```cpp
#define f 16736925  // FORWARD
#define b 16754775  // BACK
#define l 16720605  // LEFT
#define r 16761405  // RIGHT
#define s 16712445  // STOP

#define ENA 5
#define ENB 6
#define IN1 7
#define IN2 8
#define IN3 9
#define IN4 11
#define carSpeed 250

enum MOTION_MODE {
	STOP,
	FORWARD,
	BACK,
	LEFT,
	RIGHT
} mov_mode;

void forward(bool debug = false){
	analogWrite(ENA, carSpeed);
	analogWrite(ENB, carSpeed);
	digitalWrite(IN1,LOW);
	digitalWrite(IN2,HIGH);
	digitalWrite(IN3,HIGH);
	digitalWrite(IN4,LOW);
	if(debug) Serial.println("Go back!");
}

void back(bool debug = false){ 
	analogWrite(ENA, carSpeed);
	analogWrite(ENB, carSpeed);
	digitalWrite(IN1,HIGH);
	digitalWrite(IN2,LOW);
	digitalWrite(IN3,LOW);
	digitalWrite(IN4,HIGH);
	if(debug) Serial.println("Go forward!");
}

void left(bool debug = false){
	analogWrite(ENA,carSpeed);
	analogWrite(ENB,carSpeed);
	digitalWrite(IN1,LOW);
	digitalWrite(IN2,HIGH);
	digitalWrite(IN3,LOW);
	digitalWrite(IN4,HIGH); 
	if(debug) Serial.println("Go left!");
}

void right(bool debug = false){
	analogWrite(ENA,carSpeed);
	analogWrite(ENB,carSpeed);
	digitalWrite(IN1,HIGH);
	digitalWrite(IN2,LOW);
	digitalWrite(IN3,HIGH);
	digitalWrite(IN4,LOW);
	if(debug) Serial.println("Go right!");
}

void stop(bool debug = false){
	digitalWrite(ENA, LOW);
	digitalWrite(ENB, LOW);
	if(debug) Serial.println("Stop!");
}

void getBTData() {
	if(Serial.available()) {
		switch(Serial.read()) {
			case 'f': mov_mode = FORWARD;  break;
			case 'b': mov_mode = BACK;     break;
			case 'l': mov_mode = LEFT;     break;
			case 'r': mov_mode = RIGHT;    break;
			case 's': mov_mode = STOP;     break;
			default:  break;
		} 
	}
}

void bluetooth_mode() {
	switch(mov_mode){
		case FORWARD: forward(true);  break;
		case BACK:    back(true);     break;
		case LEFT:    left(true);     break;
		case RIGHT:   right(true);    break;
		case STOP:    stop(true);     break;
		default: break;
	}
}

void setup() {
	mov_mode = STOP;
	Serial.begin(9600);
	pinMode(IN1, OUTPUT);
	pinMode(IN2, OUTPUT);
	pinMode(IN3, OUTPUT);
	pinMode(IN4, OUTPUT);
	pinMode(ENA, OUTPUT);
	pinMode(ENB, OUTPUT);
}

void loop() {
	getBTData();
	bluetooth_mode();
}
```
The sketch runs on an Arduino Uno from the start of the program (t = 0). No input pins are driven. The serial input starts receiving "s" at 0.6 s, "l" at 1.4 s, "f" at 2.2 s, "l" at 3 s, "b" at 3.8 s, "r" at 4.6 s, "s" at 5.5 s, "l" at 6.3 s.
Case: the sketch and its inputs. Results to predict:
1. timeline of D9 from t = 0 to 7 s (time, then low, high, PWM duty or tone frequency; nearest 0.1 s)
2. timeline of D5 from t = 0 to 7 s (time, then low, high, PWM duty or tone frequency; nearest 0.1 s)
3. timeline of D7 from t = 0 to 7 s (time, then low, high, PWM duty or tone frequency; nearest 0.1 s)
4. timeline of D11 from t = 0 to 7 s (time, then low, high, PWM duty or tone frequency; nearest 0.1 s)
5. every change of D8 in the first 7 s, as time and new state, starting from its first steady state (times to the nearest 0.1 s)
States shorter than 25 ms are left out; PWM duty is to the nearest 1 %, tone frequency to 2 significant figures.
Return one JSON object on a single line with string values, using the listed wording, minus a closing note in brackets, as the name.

{"timeline of D9 from t = 0 to 7 s": "0 s low; 2.2 s high; 3 s low; 4.6 s high; 6.3 s low", "timeline of D5 from t = 0 to 7 s": "0 s low; 1.4 s PWM 98 %; 5.5 s low; 6.3 s PWM 98 %", "timeline of D7 from t = 0 to 7 s": "0 s low; 3.8 s high; 6.3 s low", "timeline of D11 from t = 0 to 7 s": "0 s low; 1.4 s high; 2.2 s low; 3 s high; 4.6 s low; 6.3 s high", "every change of D8 in the first 7 s, as time and new state, starting from its first steady state": "0 s low; 1.4 s high; 3.8 s low; 6.3 s high"}
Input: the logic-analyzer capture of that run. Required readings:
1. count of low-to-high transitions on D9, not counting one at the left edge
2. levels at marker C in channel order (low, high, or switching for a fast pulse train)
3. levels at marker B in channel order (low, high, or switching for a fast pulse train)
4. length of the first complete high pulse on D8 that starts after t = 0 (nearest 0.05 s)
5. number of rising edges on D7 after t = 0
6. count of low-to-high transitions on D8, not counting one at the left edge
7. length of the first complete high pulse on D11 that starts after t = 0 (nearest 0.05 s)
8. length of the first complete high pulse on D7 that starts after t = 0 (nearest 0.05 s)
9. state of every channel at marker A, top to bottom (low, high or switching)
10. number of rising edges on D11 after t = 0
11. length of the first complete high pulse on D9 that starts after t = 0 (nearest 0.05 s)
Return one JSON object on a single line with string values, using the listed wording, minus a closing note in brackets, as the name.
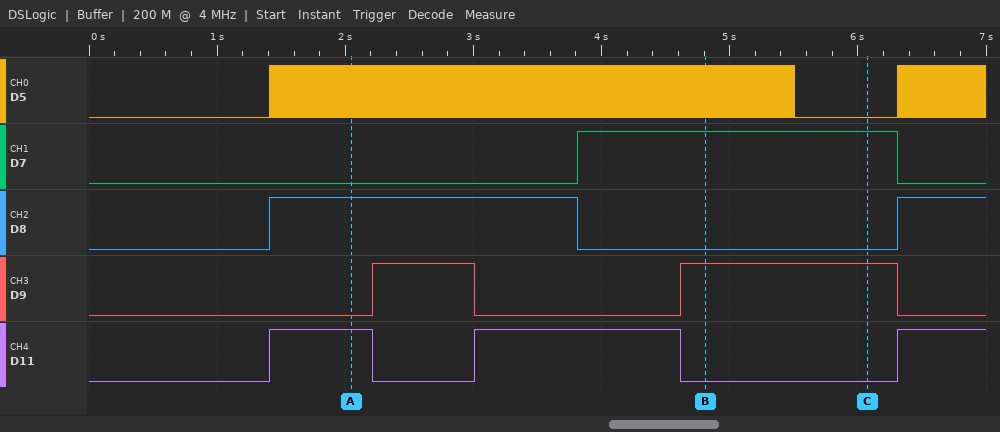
{"count of low-to-high transitions on D9, not counting one at the left edge": "2", "levels at marker C in channel order": "D5 low, D7 high, D8 low, D9 high, D11 low", "levels at marker B in channel order": "D5 switching, D7 high, D8 low, D9 high, D11 low", "length of the first complete high pulse on D8 that starts after t = 0": "2.40 s", "number of rising edges on D7 after t = 0": "1", "count of low-to-high transitions on D8, not counting one at the left edge": "2", "length of the first complete high pulse on D11 that starts after t = 0": "0.80 s", "length of the first complete high pulse on D7 that starts after t = 0": "2.50 s", "state of every channel at marker A, top to bottom": "D5 switching, D7 low, D8 high, D9 low, D11 high", "number of rising edges on D11 after t = 0": "3", "length of the first complete high pulse on D9 that starts after t = 0": "0.80 s"}
